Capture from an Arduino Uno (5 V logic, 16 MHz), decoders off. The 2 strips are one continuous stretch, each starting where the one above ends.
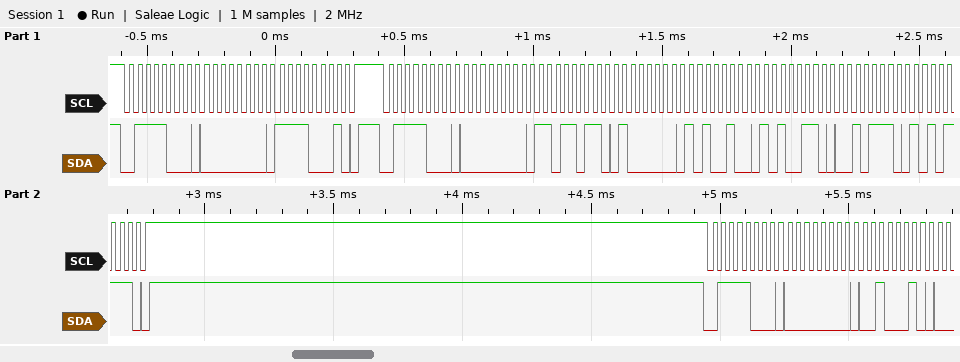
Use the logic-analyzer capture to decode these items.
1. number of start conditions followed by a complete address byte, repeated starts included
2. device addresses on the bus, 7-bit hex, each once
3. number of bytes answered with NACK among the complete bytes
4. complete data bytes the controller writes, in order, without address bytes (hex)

3
0x3C
0
00 F1 00 DB 40 A4 A6 2E AF 00 22
